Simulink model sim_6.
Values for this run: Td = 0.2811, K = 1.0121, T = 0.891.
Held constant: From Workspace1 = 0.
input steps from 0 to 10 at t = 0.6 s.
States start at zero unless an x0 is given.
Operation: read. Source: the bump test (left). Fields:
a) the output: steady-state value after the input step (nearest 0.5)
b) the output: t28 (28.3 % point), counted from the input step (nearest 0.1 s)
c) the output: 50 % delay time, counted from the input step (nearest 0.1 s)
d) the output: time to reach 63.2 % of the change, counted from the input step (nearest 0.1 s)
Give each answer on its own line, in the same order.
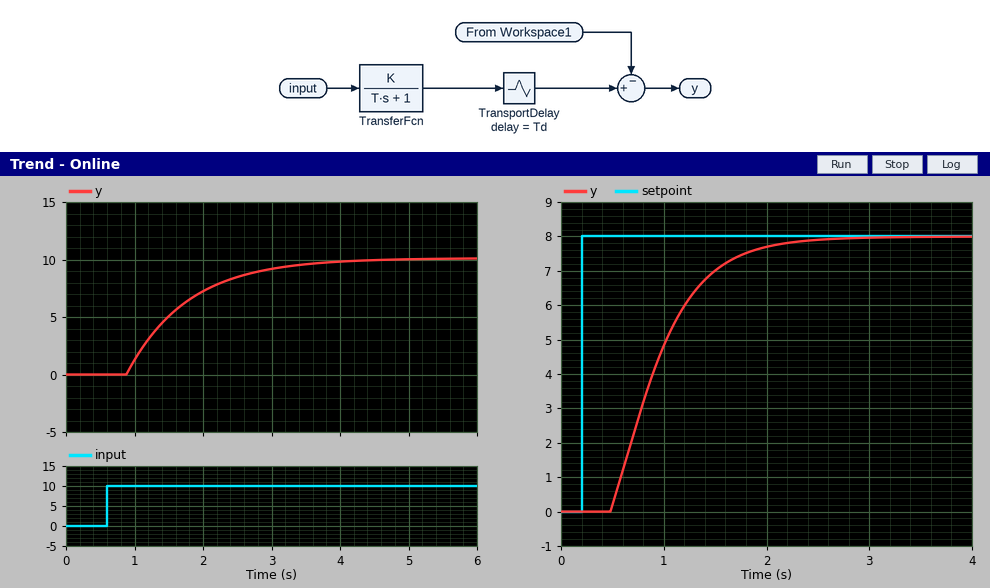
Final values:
10.0
0.6 s
0.9 s
1.2 s
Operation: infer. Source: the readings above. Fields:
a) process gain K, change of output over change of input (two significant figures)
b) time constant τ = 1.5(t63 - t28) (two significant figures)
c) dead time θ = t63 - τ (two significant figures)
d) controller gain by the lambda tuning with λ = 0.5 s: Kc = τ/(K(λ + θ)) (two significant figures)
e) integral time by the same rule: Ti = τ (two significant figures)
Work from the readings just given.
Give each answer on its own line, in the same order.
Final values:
1.0
0.90 s
0.30 s
1.1
0.90 s
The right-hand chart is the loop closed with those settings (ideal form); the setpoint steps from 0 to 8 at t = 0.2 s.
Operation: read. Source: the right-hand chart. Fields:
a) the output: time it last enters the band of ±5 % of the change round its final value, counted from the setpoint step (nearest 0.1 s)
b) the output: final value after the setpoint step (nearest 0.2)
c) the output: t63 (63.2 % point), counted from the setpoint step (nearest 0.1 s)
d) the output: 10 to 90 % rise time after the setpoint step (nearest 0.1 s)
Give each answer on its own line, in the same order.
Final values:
1.7 s
8.0
0.8 s
1.0 s
